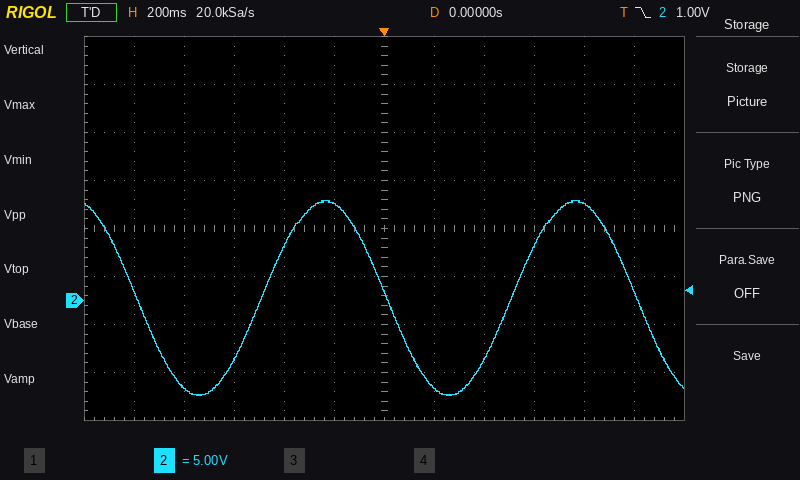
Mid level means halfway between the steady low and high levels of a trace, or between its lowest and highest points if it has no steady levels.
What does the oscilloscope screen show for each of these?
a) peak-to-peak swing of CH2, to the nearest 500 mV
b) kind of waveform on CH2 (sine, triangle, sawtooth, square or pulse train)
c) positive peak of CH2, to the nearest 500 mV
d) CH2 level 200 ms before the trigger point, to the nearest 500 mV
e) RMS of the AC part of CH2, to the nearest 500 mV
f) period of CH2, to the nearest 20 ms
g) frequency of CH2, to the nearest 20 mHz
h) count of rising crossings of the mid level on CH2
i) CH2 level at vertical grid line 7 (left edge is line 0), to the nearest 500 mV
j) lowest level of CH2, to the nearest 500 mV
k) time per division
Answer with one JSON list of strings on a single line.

["20.5 V", "sine", "10.5 V", "10.0 V", "7.0 V", "1.00 s", "1.00 Hz", "2", "-9.0 V", "-10.0 V", "200 ms"]
